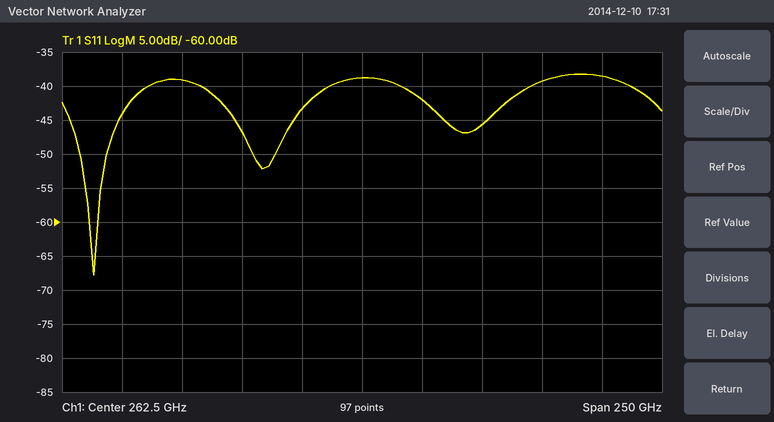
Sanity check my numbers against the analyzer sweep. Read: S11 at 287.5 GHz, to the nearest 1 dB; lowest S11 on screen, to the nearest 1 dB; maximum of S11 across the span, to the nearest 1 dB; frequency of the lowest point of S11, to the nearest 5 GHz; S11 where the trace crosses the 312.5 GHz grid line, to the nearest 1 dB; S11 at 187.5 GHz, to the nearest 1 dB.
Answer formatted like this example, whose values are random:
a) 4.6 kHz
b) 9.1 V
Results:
a) -42 dB
b) -68 dB
c) -38 dB
d) 150 GHz
e) -46 dB
f) -39 dB
